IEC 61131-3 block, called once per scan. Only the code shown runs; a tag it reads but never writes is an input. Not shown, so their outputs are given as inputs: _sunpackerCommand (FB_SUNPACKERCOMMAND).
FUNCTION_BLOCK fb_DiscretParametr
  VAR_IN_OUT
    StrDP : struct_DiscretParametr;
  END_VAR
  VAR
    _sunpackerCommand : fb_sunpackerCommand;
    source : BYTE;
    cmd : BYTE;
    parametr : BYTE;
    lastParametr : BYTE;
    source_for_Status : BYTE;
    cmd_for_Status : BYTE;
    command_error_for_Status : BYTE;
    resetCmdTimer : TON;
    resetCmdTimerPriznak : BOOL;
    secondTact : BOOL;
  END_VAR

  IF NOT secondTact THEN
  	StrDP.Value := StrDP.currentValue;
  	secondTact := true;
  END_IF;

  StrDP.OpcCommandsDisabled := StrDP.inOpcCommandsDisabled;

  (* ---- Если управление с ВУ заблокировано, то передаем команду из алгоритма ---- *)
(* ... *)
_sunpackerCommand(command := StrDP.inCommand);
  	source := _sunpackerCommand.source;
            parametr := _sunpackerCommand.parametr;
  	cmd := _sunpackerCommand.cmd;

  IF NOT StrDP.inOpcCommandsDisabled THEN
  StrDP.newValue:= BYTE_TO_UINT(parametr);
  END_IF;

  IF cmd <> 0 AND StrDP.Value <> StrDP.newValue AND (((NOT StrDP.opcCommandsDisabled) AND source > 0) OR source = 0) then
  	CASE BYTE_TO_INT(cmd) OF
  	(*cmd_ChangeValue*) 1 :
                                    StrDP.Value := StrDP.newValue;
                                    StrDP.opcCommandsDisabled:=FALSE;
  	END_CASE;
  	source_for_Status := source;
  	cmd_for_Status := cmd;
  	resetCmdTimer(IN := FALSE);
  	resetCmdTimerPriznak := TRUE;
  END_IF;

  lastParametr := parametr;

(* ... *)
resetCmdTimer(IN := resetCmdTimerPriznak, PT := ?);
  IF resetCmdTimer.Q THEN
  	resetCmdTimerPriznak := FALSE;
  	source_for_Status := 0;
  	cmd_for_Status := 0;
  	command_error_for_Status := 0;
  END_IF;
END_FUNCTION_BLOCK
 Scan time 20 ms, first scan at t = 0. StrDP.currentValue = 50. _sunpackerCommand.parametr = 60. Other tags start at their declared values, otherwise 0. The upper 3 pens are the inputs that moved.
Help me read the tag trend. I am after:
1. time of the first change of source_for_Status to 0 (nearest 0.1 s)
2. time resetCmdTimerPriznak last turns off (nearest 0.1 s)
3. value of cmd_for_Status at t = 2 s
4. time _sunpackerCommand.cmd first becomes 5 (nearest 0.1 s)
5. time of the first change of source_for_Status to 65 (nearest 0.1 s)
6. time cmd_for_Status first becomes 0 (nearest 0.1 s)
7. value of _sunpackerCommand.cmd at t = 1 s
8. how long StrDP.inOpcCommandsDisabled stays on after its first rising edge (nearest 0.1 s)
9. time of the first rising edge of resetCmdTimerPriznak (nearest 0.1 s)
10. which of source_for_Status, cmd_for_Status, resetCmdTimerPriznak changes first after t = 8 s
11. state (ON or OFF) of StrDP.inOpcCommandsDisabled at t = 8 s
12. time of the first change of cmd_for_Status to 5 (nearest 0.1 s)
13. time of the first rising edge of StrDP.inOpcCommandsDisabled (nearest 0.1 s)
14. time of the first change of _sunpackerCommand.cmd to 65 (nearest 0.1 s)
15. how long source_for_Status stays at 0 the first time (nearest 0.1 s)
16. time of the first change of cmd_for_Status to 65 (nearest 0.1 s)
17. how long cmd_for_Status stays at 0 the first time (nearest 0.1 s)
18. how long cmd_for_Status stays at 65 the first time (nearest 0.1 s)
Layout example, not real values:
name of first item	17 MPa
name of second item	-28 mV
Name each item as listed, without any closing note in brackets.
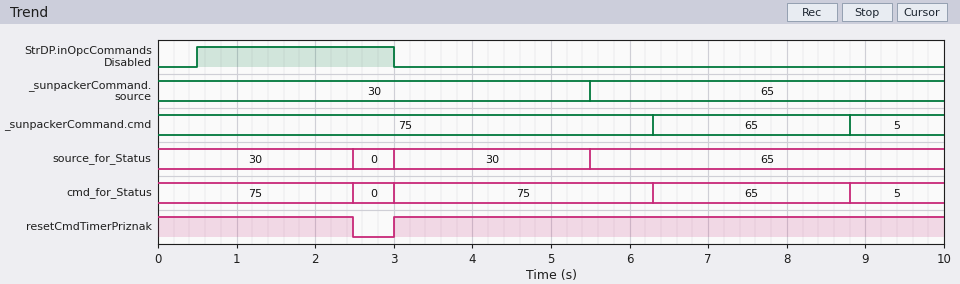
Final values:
time of the first change of source_for_Status to 0	2.5 s
time resetCmdTimerPriznak last turns off	2.5 s
value of cmd_for_Status at t = 2 s	75
time _sunpackerCommand.cmd first becomes 5	8.8 s
time of the first change of source_for_Status to 65	5.5 s
time cmd_for_Status first becomes 0	2.5 s
value of _sunpackerCommand.cmd at t = 1 s	75
how long StrDP.inOpcCommandsDisabled stays on after its first rising edge	2.5 s
time of the first rising edge of resetCmdTimerPriznak	3.0 s
which of source_for_Status, cmd_for_Status, resetCmdTimerPriznak changes first after t = 8 s	cmd_for_Status
state (ON or OFF) of StrDP.inOpcCommandsDisabled at t = 8 s	OFF
time of the first change of cmd_for_Status to 5	8.8 s
time of the first rising edge of StrDP.inOpcCommandsDisabled	0.5 s
time of the first change of _sunpackerCommand.cmd to 65	6.3 s
how long source_for_Status stays at 0 the first time	0.5 s
time of the first change of cmd_for_Status to 65	6.3 s
how long cmd_for_Status stays at 0 the first time	0.5 s
how long cmd_for_Status stays at 65 the first time	2.5 s
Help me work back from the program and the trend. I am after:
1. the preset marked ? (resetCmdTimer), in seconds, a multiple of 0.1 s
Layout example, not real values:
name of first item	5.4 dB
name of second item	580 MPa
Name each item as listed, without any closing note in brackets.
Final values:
the preset marked ? (resetCmdTimer), in seconds, a multiple of 0.1 s	2.0 s
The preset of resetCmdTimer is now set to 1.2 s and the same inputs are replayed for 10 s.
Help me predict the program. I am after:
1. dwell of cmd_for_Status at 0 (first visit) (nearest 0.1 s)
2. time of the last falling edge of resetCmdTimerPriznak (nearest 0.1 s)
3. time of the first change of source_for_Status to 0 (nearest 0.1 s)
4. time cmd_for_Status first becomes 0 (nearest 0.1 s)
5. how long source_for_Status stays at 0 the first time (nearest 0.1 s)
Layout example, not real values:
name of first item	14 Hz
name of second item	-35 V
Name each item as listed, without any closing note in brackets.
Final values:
dwell of cmd_for_Status at 0 (first visit)	1.3 s
time of the last falling edge of resetCmdTimerPriznak	1.7 s
time of the first change of source_for_Status to 0	1.7 s
time cmd_for_Status first becomes 0	1.7 s
how long source_for_Status stays at 0 the first time	1.3 s
